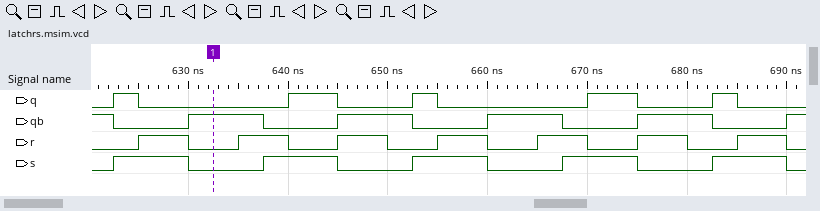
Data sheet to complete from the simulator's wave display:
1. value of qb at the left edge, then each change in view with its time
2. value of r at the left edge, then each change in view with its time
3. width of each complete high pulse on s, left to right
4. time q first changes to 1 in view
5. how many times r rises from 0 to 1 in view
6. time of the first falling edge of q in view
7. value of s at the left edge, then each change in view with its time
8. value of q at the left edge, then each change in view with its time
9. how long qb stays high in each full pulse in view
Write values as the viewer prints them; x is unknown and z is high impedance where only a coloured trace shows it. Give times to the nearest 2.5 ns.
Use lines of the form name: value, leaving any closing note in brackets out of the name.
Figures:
value of qb at the left edge, then each change in view with its time: 1, 0 at 622.5 ns, 1 at 630 ns, 0 at 637.5 ns, 1 at 645 ns, 0 at 652.5 ns, 1 at 660 ns, 0 at 667.5 ns, 1 at 675 ns, 0 at 682.5 ns, 1 at 690 ns
value of r at the left edge, then each change in view with its time: 0, 1 at 625 ns, 0 at 630 ns, 1 at 635 ns, 0 at 640 ns, 1 at 645 ns, 0 at 650 ns, 1 at 655 ns, 0 at 660 ns, 1 at 665 ns, 0 at 670 ns, 1 at 675 ns, 0 at 680 ns, 1 at 685 ns, 0 at 690 ns
width of each complete high pulse on s, left to right: 7.5 ns, 7.5 ns, 7.5 ns, 7.5 ns, 7.5 ns
time q first changes to 1 in view: 622.5 ns
how many times r rises from 0 to 1 in view: 7
time of the first falling edge of q in view: 625 ns
value of s at the left edge, then each change in view with its time: 0, 1 at 622.5 ns, 0 at 630 ns, 1 at 637.5 ns, 0 at 645 ns, 1 at 652.5 ns, 0 at 660 ns, 1 at 667.5 ns, 0 at 675 ns, 1 at 682.5 ns, 0 at 690 ns
value of q at the left edge, then each change in view with its time: 0, 1 at 622.5 ns, 0 at 625 ns, 1 at 640 ns, 0 at 645 ns, 1 at 652.5 ns, 0 at 655 ns, 1 at 670 ns, 0 at 675 ns, 1 at 682.5 ns, 0 at 685 ns
how long qb stays high in each full pulse in view: 7.5 ns, 7.5 ns, 7.5 ns, 7.5 ns
